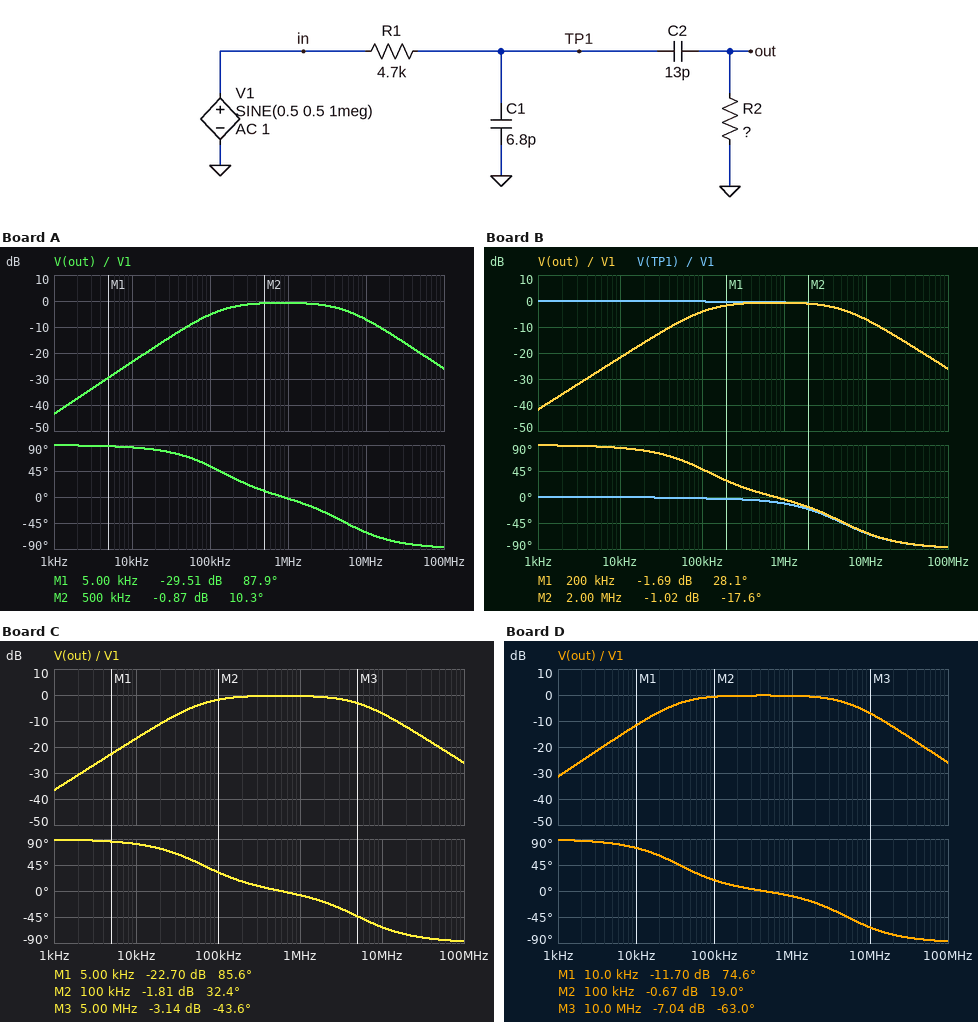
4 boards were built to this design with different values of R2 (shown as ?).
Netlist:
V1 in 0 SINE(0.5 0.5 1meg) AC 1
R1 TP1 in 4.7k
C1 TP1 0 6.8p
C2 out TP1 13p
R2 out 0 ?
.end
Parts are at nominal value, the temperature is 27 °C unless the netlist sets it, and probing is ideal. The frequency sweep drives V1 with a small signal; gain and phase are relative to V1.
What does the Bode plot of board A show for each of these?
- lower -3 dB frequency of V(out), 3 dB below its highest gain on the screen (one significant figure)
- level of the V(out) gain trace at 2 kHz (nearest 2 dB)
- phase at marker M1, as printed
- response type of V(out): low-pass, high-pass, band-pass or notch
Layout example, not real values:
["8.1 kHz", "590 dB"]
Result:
["100 kHz", "-38 dB", "87.9 deg", "band-pass"]
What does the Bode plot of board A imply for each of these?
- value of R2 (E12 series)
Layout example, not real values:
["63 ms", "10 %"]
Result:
["82 kΩ"]
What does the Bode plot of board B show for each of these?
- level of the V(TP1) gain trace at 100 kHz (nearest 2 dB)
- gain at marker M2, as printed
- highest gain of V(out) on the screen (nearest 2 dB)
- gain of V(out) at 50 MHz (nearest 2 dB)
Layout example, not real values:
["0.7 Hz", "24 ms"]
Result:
["0 dB", "-1.02 dB", "0 dB", "-20 dB"]
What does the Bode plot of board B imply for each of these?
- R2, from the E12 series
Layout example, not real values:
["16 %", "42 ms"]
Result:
["100 kΩ"]
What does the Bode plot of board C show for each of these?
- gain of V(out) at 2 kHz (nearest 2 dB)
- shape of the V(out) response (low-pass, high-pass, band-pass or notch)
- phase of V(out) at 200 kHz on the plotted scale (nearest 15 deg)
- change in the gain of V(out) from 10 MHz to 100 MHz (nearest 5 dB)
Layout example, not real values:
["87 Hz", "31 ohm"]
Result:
["-30 dB", "band-pass", "15 deg", "-20 dB"]
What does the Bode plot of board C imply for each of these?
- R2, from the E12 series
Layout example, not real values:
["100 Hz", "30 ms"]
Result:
["180 kΩ"]
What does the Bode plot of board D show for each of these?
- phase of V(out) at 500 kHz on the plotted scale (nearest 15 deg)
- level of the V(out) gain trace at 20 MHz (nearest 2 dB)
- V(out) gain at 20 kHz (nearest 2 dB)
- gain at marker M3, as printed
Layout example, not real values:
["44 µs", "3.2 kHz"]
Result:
["0 deg", "-12 dB", "-6 dB", "-7.04 dB"]
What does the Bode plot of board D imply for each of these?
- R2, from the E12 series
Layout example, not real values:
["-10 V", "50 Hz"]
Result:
["330 kΩ"]
